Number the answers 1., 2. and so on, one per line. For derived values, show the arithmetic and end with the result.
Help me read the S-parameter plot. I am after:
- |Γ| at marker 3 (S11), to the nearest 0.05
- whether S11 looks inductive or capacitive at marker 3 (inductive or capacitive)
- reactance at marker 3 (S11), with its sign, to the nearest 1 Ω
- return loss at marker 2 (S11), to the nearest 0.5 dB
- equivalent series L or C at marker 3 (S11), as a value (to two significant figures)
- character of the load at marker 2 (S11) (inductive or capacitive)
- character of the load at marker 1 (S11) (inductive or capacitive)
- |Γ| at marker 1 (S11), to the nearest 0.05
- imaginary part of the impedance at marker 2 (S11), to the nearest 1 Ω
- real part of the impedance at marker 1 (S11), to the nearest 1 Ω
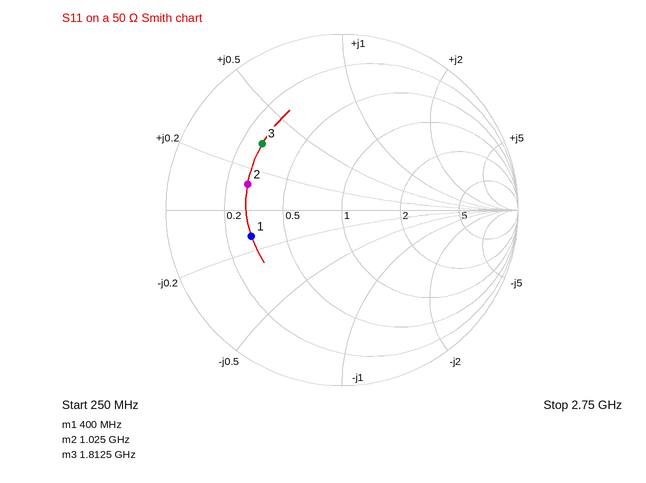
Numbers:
1. 0.60
2. inductive
3. +17 Ω
4. 5.0 dB
5. L = 17 Ω/(2π × 1.8125 GHz) ≈ 1.5 nH
6. inductive
7. capacitive
8. 0.55
9. +6 Ω
10. 15 Ω
